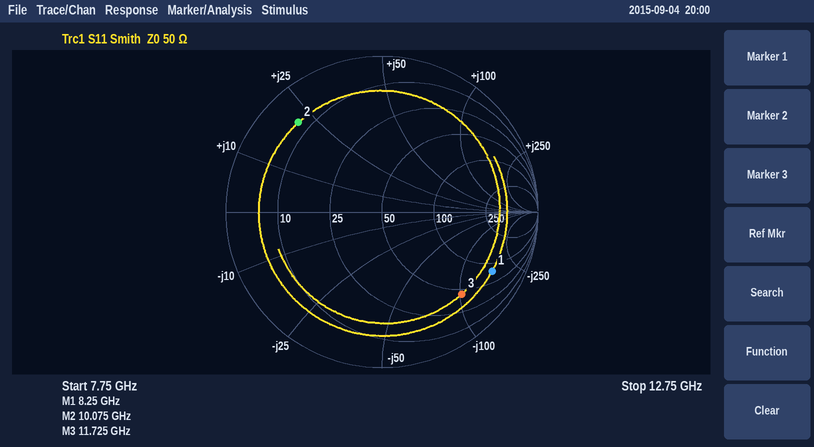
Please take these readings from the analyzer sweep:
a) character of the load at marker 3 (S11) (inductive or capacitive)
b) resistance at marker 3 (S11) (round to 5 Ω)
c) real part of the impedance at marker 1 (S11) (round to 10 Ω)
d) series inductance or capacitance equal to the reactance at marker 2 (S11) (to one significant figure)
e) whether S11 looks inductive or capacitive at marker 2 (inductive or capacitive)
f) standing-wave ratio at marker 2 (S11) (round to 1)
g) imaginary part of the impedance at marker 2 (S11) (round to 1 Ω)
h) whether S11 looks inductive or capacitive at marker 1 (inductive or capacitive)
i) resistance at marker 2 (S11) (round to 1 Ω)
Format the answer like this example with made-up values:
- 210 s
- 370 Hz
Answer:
- capacitive
- 45 Ω
- 80 Ω
- 300 pH
- inductive
- 8
- +21 Ω
- capacitive
- 7 Ω
